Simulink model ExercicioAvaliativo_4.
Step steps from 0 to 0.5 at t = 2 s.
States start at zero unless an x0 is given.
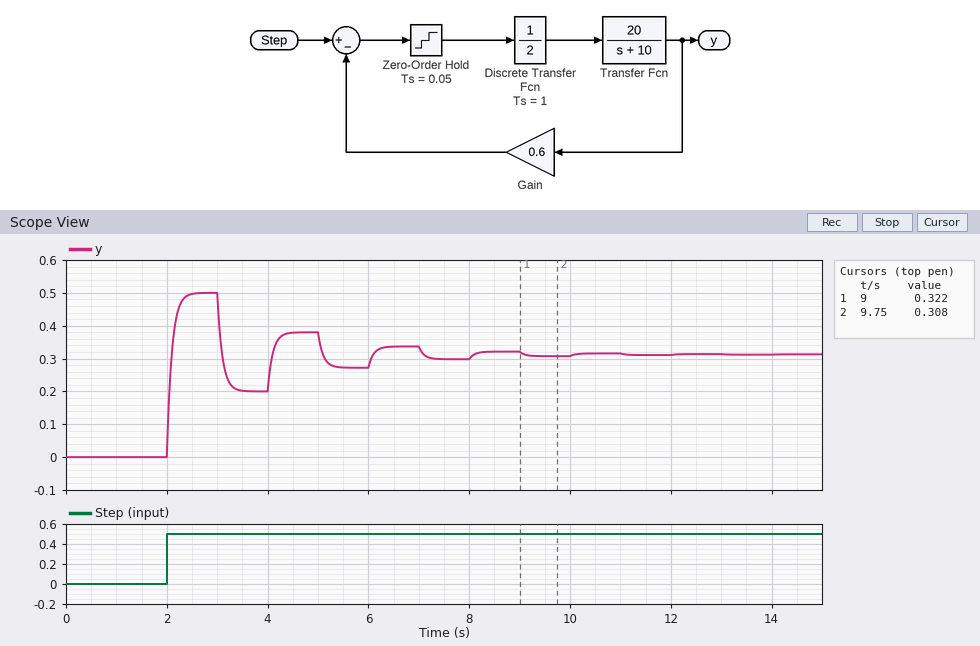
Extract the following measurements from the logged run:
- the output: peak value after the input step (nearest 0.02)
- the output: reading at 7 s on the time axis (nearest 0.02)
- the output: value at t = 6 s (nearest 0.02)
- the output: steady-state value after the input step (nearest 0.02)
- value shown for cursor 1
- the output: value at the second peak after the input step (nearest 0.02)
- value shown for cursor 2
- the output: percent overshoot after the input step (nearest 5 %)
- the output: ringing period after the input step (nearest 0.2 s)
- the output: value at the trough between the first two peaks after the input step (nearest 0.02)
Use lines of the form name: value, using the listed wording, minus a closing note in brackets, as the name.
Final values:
the output: peak value after the input step: 0.50
the output: reading at 7 s on the time axis: 0.34
the output: value at t = 6 s: 0.28
the output: steady-state value after the input step: 0.32
value shown for cursor 1: 0.322
the output: value at the second peak after the input step: 0.38
value shown for cursor 2: 0.308
the output: percent overshoot after the input step: 60 %
the output: ringing period after the input step: 2.0 s
the output: value at the trough between the first two peaks after the input step: 0.20
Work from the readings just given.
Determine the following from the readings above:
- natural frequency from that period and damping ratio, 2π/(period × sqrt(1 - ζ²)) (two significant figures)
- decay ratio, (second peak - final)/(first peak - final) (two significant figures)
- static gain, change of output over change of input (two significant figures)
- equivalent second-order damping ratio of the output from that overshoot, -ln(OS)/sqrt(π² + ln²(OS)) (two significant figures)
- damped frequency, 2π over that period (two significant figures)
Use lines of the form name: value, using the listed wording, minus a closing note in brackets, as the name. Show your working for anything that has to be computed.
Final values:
natural frequency from that period and damping ratio, 2π/(period × sqrt(1 - ζ²)): 2π / (2 × sqrt(1 - 0.16²)) = 3.2 rad/s
decay ratio, (second peak - final)/(first peak - final): (0.38 - 0.32) / (0.5 - 0.32) = 0.33
static gain, change of output over change of input: (0.32 - 0) / (0.5 - 0) = 0.64
equivalent second-order damping ratio of the output from that overshoot, -ln(OS)/sqrt(π² + ln²(OS)): ln(0.6) = -0.511; 0.511 / sqrt(9.870 + 0.261) = 0.16
damped frequency, 2π over that period: 2π / 2 = 3.1 rad/s
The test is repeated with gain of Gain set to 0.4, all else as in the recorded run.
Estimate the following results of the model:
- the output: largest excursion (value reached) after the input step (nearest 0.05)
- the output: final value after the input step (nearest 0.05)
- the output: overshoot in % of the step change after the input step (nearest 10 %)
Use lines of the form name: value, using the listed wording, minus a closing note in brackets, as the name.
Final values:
the output: largest excursion (value reached) after the input step: 0.50
the output: final value after the input step: 0.35
the output: overshoot in % of the step change after the input step: 40 %
